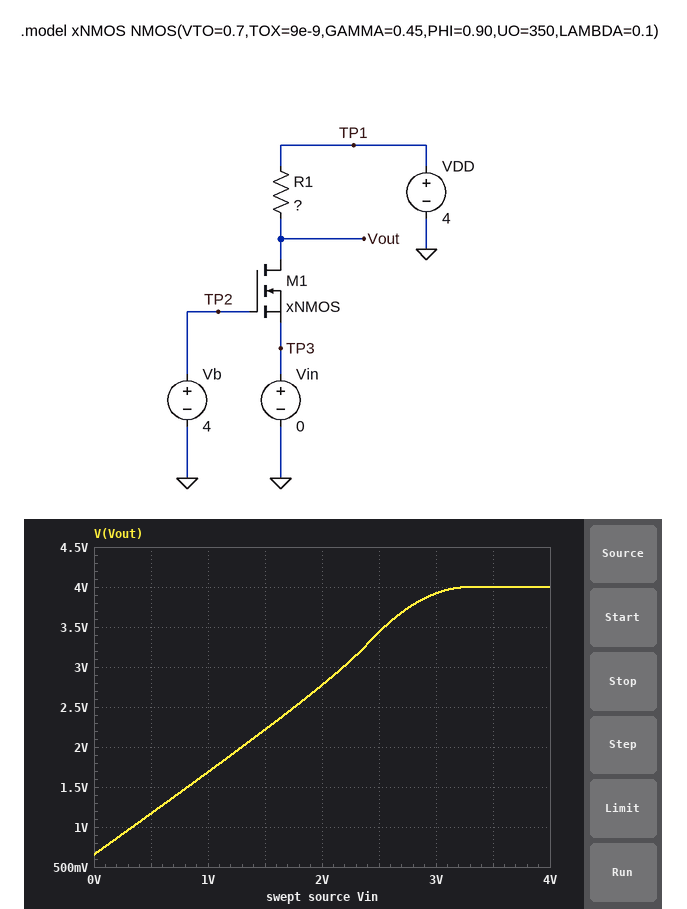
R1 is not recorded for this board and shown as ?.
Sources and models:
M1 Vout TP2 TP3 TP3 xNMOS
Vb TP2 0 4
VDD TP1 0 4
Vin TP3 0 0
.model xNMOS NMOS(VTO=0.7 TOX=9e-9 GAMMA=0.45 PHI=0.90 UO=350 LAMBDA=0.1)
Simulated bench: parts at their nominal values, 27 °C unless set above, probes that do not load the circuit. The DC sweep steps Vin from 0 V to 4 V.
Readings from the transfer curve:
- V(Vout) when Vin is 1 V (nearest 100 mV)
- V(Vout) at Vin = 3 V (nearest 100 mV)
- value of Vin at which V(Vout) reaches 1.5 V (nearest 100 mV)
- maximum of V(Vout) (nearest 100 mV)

1.7 V
3.9 V
800 mV
4.0 V
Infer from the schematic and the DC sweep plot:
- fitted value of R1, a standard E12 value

12 kΩ
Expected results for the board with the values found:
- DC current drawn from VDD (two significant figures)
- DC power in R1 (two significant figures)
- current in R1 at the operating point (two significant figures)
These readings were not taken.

280 µA
930 µW
280 µA
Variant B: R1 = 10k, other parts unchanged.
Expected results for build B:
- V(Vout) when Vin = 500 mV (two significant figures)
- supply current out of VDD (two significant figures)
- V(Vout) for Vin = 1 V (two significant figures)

1.3 V
320 µA
1.8 V
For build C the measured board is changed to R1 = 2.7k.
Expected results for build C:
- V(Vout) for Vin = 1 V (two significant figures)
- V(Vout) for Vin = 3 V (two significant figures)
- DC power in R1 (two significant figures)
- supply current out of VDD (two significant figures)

2.9 V
4.0 V
1.5 mW
740 µA
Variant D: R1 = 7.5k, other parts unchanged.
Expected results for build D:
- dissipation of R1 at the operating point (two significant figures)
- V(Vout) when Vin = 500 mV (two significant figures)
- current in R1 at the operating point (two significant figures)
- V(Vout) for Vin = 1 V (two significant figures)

1.2 mW
1.5 V
400 µA
2.0 V
